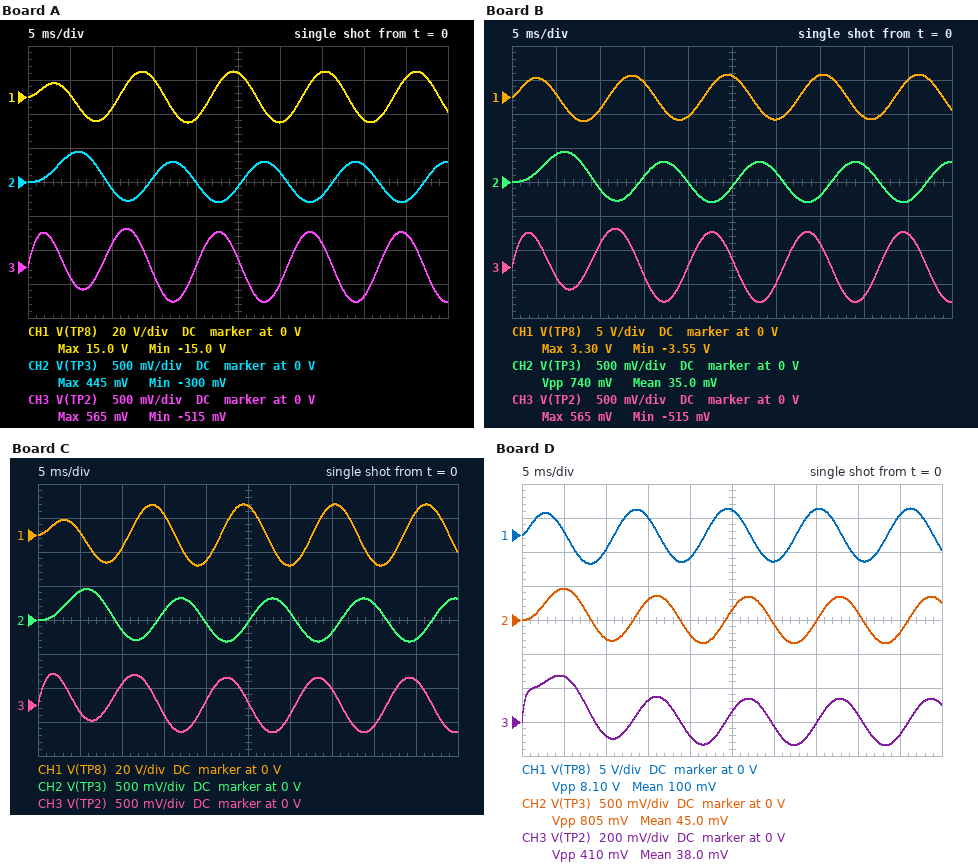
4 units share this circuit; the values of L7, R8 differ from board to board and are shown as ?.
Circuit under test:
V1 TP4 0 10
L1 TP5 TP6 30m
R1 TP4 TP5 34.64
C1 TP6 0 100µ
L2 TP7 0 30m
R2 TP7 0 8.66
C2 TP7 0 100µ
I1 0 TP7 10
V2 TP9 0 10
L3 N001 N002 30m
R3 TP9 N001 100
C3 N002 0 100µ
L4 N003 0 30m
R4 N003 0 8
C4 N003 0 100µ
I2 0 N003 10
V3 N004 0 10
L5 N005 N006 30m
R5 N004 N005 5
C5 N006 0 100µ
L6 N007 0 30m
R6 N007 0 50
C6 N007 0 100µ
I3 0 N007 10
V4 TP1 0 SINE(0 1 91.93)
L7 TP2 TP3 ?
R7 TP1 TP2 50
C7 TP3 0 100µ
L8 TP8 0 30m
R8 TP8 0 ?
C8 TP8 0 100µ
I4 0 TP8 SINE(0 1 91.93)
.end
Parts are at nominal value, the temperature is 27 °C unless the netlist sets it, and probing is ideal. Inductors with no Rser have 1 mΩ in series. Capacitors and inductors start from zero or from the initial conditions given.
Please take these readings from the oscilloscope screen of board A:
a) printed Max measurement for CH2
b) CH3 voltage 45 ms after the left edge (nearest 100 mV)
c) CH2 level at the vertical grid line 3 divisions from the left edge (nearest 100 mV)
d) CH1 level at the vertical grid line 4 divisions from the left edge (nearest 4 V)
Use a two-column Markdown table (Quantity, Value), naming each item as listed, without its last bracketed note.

| Quantity | Value |
|---|---|
| printed Max measurement for CH2 | 445 mV |
| CH3 voltage 45 ms after the left edge | 500 mV |
| CH2 level at the vertical grid line 3 divisions from the left edge | 100 mV |
| CH1 level at the vertical grid line 4 divisions from the left edge | -12 V |
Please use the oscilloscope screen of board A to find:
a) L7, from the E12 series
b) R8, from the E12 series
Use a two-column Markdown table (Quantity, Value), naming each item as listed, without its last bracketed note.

| Quantity | Value |
|---|---|
| L7, from the E12 series | 82 mH |
| R8, from the E12 series | 15 Ω |
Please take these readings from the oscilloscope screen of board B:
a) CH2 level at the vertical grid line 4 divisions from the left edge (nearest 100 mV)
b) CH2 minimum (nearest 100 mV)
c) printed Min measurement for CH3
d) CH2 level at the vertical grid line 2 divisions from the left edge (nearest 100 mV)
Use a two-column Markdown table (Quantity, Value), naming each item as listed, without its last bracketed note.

| Quantity | Value |
|---|---|
| CH2 level at the vertical grid line 4 divisions from the left edge | 0 V |
| CH2 minimum | -300 mV |
| printed Min measurement for CH3 | -515 mV |
| CH2 level at the vertical grid line 2 divisions from the left edge | -100 mV |
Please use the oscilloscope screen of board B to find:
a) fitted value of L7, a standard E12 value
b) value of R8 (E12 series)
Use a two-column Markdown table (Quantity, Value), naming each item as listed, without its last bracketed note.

| Quantity | Value |
|---|---|
| fitted value of L7, a standard E12 value | 82 mH |
| value of R8 | 3.3 Ω |
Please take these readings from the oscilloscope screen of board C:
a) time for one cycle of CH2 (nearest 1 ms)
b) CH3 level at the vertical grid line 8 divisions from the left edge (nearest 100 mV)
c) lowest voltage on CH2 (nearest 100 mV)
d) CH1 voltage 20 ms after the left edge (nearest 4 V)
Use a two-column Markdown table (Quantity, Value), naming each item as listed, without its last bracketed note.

| Quantity | Value |
|---|---|
| time for one cycle of CH2 | 11 ms |
| CH3 level at the vertical grid line 8 divisions from the left edge | -300 mV |
| lowest voltage on CH2 | -300 mV |
| CH1 voltage 20 ms after the left edge | -16 V |
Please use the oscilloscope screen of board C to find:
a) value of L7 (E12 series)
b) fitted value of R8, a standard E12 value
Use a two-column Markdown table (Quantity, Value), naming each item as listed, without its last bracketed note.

| Quantity | Value |
|---|---|
| value of L7 | 68 mH |
| fitted value of R8, a standard E12 value | 18 Ω |
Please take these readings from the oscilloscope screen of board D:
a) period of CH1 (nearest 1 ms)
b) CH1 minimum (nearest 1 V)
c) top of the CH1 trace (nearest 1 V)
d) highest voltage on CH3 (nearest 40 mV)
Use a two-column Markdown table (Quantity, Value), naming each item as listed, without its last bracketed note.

| Quantity | Value |
|---|---|
| period of CH1 | 11 ms |
| CH1 minimum | -4 V |
| top of the CH1 trace | 4 V |
| highest voltage on CH3 | 280 mV |
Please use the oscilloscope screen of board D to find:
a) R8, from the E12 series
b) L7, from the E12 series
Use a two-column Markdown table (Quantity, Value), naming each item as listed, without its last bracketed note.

| Quantity | Value |
|---|---|
| R8, from the E12 series | 3.9 Ω |
| L7, from the E12 series | 18 mH |
